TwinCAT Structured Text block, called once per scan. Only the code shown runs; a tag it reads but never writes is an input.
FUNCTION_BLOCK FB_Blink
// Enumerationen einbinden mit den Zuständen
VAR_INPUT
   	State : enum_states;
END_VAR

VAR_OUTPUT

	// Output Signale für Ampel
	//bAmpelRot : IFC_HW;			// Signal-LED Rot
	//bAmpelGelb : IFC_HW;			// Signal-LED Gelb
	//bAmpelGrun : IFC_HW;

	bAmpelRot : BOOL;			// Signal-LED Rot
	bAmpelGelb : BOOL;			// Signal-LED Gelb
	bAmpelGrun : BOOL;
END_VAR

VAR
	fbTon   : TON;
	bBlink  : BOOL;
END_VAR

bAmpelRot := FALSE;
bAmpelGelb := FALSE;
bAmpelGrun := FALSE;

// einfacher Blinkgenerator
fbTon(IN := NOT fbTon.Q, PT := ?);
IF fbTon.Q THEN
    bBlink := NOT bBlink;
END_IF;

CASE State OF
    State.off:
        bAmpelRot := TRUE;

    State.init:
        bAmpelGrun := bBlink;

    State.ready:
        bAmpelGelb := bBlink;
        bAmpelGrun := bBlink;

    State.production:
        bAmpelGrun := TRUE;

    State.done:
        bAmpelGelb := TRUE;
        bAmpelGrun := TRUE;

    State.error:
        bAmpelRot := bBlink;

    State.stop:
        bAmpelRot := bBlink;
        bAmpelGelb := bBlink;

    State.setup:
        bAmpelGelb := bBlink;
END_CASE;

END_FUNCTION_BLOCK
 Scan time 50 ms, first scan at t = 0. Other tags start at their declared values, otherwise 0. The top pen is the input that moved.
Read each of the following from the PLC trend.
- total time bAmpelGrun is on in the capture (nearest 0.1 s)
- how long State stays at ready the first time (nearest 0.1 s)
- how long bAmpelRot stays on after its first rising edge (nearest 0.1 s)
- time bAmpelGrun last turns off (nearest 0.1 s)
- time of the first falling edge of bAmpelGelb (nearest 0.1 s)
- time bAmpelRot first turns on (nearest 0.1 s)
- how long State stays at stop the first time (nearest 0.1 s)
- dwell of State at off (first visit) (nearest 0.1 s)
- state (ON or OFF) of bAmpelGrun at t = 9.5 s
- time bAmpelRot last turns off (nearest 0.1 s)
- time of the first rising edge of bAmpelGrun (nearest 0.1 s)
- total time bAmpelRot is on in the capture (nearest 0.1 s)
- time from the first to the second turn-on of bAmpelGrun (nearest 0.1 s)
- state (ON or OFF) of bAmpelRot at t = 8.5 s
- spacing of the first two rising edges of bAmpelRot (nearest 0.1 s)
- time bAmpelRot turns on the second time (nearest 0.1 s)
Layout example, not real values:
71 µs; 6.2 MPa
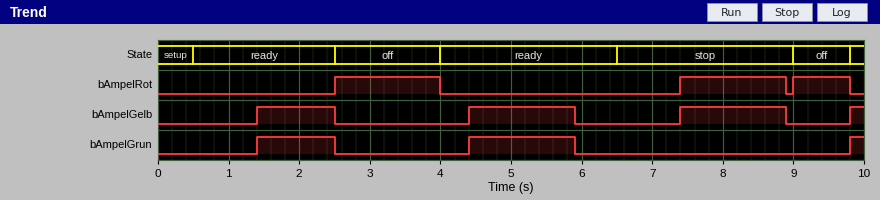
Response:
2.8 s; 2.0 s; 1.5 s; 5.9 s; 2.5 s; 2.5 s; 2.5 s; 1.5 s; OFF; 9.8 s; 1.4 s; 3.8 s; 3.0 s; ON; 4.9 s; 7.4 s
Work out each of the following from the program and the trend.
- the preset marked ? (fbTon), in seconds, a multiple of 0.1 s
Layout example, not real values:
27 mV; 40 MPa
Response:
1.4 s
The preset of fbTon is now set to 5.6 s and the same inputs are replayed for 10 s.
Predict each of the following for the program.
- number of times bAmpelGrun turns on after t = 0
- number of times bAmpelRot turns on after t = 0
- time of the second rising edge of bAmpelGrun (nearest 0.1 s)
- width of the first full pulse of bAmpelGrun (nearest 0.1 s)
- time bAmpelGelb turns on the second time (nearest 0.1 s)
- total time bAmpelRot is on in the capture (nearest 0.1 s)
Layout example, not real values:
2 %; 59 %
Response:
2; 2; 9.8 s; 0.9 s; 9.8 s; 4.8 s
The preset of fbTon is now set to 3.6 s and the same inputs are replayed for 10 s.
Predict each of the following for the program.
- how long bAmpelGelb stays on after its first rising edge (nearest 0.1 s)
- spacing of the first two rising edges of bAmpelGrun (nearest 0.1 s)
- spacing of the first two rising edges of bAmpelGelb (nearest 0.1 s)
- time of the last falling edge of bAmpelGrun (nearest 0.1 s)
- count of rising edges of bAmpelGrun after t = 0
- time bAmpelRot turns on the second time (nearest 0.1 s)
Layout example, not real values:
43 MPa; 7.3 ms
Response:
3.3 s; 5.8 s; 5.8 s; 6.5 s; 2; 6.5 s
